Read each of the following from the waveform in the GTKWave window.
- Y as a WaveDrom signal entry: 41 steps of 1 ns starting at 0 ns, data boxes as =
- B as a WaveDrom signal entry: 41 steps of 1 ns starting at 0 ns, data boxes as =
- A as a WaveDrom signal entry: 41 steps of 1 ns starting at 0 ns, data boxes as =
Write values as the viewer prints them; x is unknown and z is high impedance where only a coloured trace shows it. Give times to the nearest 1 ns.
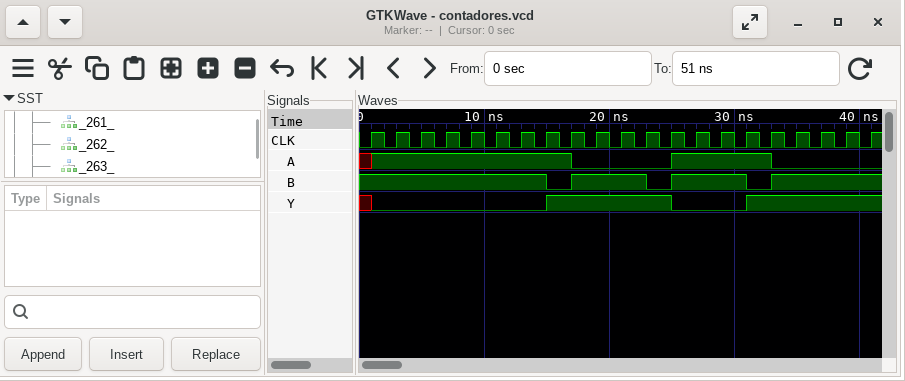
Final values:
{name: 'Y', wave: 'x0.............1.........0.....1.........'}
{name: 'B', wave: '1..............0.1.....0.1.....0.1.......'}
{name: 'A', wave: 'x1...............0.......1.......0.......'}
